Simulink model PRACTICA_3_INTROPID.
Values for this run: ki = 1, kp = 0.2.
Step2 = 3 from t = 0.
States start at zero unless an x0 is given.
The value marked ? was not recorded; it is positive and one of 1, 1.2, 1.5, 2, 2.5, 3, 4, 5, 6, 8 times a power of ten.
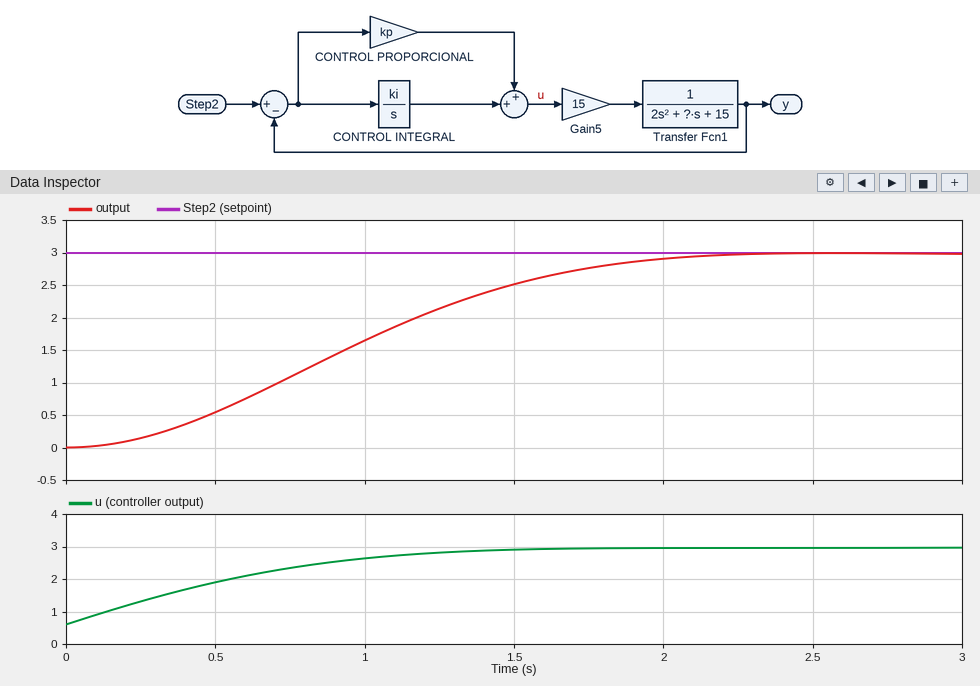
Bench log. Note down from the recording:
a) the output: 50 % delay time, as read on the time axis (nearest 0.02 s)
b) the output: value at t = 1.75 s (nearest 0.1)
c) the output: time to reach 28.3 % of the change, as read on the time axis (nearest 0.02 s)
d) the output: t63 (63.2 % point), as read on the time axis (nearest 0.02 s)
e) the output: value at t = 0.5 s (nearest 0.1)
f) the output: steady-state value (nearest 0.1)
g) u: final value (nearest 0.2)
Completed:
0.94 s
2.8
0.64 s
1.12 s
0.5
3.0
3.0
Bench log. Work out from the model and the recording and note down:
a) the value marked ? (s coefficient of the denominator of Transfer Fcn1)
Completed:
8
